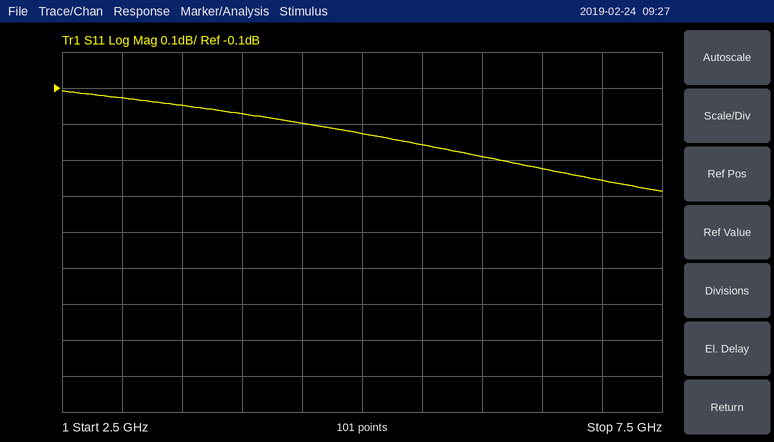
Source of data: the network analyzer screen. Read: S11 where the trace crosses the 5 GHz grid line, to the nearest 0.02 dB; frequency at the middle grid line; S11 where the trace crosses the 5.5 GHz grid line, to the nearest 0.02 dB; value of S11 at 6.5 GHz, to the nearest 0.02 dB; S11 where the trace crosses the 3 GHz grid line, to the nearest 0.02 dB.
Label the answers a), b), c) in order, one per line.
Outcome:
a) -0.22 dB
b) 5 GHz
c) -0.26 dB
d) -0.32 dB
e) -0.12 dB
